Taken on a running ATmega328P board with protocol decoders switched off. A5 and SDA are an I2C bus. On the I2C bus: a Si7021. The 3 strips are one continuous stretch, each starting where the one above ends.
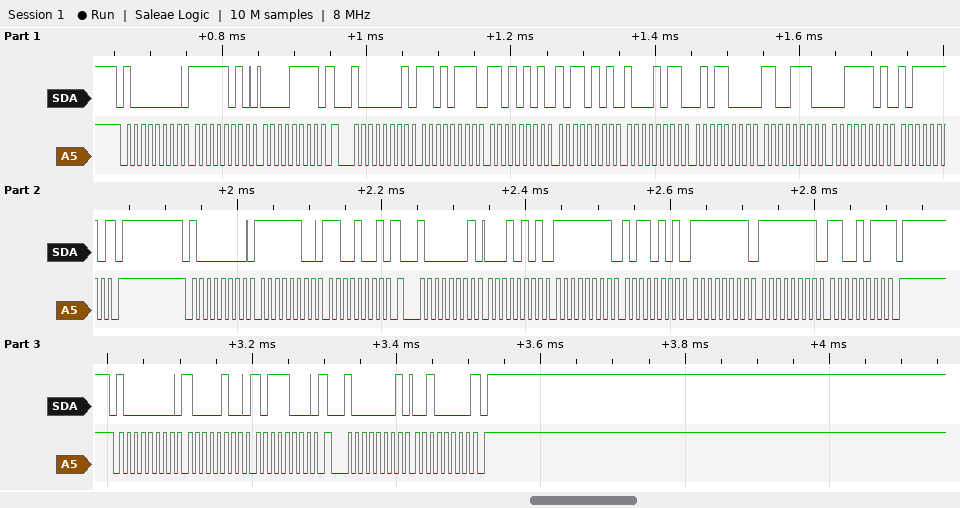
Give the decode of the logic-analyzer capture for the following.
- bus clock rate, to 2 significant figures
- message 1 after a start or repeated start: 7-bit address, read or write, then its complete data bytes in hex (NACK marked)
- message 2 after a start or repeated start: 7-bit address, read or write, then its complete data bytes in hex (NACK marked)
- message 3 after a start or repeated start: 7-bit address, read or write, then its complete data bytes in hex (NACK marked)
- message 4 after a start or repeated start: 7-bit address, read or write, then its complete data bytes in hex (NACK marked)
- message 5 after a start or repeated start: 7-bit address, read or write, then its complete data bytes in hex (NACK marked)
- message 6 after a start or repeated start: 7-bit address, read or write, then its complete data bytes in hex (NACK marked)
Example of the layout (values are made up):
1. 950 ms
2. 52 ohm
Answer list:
1. 100 kHz
2. 0x40 write: FA 0F
3. 0x40 read: D7 D5 B5 8B 58 CE 3D BE NACK
4. 0x40 write: FC C9
5. 0x40 read: 15 FF B5 FF FF CB NACK
6. 0x40 write: 84 B8
7. 0x40 read: 20 NACK
